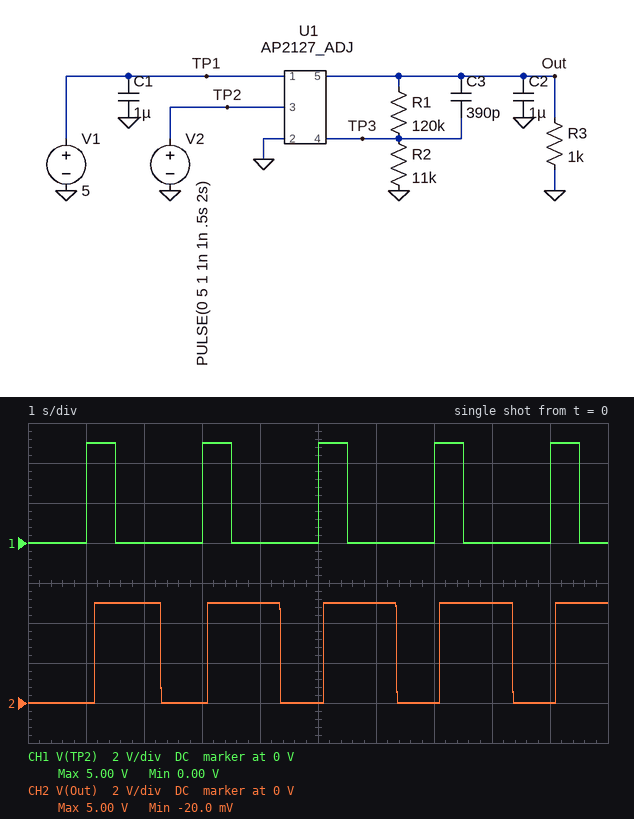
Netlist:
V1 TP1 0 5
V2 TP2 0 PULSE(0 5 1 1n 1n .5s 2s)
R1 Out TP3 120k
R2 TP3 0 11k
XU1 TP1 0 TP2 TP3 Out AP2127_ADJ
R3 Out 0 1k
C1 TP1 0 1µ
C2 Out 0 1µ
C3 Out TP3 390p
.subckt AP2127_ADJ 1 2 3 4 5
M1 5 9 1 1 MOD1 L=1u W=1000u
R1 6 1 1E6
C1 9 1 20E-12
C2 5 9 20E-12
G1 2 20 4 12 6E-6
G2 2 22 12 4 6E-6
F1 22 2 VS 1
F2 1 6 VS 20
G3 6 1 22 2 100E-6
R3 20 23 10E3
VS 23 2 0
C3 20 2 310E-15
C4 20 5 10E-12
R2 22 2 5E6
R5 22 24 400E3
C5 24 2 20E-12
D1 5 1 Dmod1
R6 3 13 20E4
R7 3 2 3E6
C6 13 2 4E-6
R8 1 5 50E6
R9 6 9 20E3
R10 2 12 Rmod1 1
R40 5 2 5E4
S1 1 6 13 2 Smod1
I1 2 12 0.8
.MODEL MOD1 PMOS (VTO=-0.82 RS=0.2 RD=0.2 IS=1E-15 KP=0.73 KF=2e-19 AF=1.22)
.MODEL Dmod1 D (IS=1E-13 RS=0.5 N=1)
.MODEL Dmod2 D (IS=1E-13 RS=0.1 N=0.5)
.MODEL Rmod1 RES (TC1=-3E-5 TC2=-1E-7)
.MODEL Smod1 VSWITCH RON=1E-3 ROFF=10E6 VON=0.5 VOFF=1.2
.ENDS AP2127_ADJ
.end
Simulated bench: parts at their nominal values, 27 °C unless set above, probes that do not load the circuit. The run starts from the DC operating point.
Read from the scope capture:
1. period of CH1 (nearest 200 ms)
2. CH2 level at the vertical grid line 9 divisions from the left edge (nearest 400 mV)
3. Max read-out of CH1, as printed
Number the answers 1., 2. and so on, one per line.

1. 2.0 s
2. 0 V
3. 5.00 V
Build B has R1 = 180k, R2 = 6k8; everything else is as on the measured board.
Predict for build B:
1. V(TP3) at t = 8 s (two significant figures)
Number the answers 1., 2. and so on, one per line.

1. 180 mV
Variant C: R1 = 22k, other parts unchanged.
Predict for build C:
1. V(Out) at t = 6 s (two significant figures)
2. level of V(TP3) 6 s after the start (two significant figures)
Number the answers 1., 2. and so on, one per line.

1. 2.4 V
2. 800 mV
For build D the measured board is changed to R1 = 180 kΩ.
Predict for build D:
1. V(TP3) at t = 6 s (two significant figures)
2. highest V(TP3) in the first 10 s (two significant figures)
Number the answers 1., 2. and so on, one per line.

1. 290 mV
2. 300 mV
